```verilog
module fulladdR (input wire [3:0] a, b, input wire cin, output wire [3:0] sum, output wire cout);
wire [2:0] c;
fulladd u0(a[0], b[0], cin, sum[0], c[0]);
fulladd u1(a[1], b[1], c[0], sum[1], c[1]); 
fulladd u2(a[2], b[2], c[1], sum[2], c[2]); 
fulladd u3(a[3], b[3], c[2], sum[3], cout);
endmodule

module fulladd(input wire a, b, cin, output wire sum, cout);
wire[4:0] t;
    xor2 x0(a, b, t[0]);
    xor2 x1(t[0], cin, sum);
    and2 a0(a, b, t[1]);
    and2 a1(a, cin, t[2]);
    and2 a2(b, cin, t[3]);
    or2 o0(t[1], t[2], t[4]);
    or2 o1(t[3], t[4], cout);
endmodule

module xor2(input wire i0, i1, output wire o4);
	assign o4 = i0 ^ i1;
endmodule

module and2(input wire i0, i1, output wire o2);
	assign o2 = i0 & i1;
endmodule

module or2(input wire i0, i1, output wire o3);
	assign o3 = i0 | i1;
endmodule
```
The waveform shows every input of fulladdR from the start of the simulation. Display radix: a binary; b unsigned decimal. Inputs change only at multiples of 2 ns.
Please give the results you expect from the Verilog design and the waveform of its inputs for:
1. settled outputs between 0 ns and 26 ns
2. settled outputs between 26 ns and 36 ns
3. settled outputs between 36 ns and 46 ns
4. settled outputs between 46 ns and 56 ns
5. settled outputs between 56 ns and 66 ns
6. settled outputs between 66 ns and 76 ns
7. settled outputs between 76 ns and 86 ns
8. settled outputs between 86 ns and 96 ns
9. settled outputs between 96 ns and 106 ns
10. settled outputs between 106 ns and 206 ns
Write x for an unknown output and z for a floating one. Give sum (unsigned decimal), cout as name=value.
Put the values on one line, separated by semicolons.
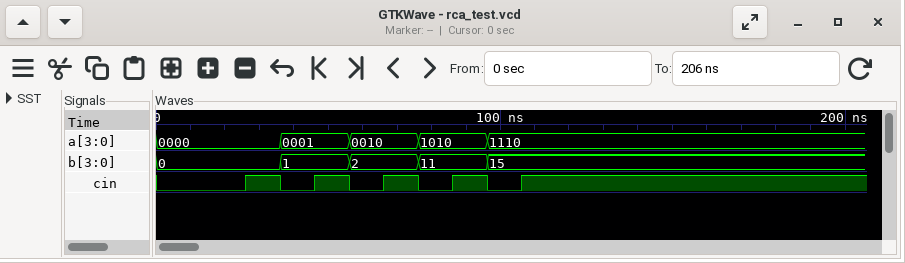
sum=0, cout=0; sum=1, cout=0; sum=2, cout=0; sum=3, cout=0; sum=4, cout=0; sum=5, cout=0; sum=5, cout=1; sum=6, cout=1; sum=13, cout=1; sum=14, cout=1
